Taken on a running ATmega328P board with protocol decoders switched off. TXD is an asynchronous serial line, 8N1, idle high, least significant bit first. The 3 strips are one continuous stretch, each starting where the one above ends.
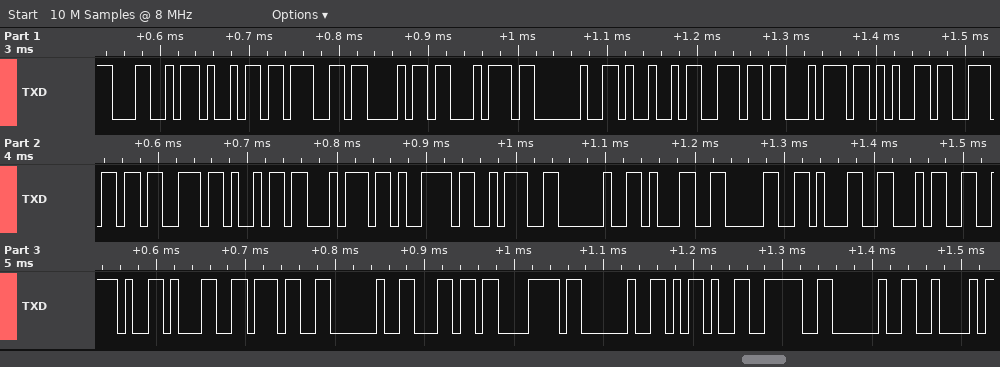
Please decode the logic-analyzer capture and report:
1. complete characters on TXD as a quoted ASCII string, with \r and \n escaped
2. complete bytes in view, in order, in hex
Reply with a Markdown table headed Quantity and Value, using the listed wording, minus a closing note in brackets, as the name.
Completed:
| Quantity | Value |
|---|---|
| complete characters on TXD as a quoted ASCII string, with \r and \n escaped | "Light Intensity: 1014.17 lx -> B" |
| complete bytes in view, in order, in hex | 4C 69 67 68 74 20 49 6E 74 65 6E 73 69 74 79 3A 20 31 30 31 34 2E 31 37 20 6C 78 20 2D 3E 20 42 |
